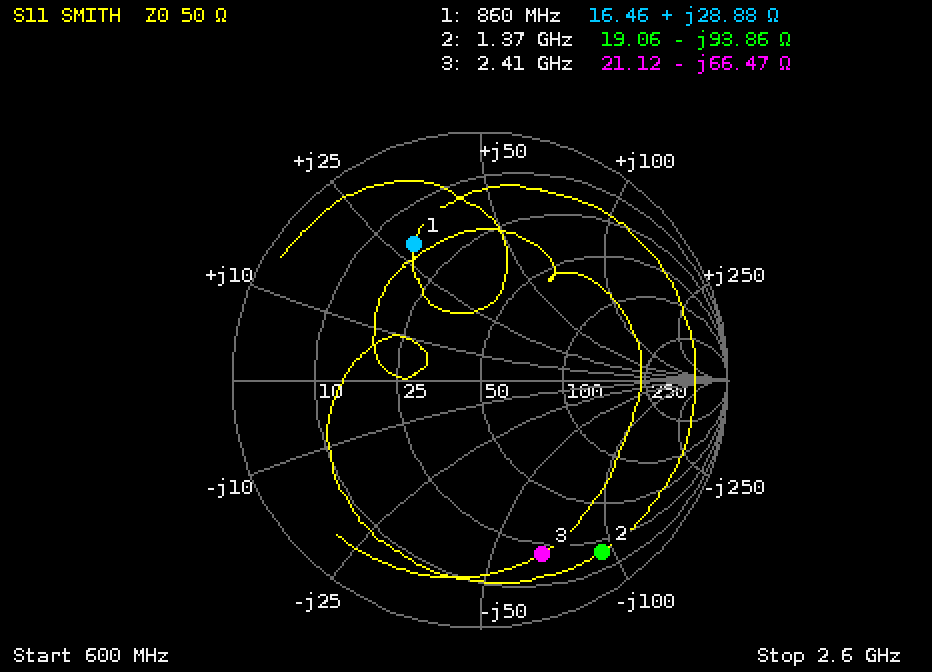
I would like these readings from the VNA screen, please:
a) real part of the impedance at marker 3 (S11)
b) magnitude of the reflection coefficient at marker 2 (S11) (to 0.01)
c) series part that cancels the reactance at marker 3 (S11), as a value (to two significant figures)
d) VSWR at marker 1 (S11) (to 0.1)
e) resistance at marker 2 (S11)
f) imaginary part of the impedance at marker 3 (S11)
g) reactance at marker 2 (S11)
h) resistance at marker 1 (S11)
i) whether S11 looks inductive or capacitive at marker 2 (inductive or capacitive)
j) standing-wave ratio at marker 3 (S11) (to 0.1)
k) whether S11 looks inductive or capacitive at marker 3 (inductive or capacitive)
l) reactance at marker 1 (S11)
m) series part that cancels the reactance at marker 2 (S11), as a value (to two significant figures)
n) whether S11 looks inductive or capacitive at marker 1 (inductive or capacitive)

21.12 Ω
0.85
4.4 nH
4.1
19.06 Ω
-66.47 Ω
-93.86 Ω
16.46 Ω
capacitive
6.8
capacitive
+28.88 Ω
11 nH
inductive
